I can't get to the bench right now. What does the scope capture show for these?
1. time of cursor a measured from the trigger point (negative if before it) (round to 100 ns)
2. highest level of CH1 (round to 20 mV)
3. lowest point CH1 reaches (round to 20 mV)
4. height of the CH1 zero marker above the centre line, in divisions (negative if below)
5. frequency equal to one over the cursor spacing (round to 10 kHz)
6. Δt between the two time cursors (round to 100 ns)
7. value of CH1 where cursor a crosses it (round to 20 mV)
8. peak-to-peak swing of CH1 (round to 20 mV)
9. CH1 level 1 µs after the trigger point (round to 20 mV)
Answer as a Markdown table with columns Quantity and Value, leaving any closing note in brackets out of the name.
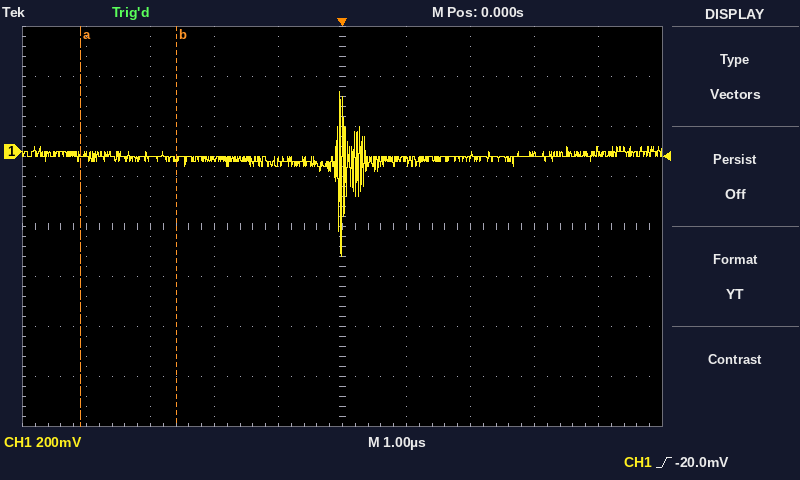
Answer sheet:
| Quantity | Value |
|---|---|
| time of cursor a measured from the trigger point (negative if before it) | -4.1 µs |
| highest level of CH1 | 240 mV |
| lowest point CH1 reaches | -420 mV |
| height of the CH1 zero marker above the centre line, in divisions | +1.5 div |
| frequency equal to one over the cursor spacing | 670 kHz |
| Δt between the two time cursors | 1.5 µs |
| value of CH1 where cursor a crosses it | -20 mV |
| peak-to-peak swing of CH1 | 660 mV |
| CH1 level 1 µs after the trigger point | -40 mV |
